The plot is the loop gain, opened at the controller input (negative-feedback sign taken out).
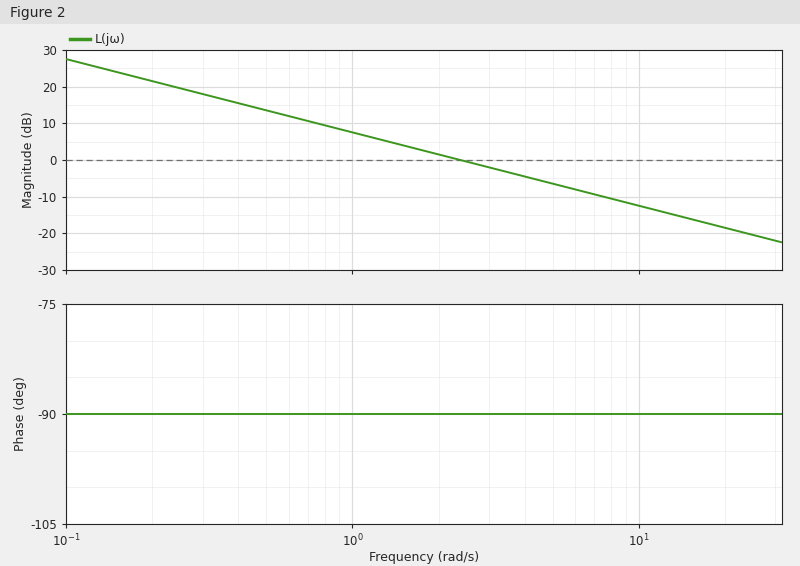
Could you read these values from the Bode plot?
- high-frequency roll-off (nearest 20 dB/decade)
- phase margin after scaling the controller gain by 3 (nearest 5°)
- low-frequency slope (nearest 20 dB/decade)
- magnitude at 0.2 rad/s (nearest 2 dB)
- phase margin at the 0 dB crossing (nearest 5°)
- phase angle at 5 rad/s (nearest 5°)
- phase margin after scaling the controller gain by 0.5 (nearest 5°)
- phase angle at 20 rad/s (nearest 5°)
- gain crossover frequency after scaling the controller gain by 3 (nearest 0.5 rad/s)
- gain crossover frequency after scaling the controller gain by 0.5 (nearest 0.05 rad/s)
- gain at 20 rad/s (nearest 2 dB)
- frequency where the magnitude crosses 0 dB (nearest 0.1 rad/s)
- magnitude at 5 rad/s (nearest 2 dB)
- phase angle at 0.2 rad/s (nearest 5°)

-20 dB/decade
90°
-20 dB/decade
22 dB
90°
-90°
90°
-90°
7.0 rad/s
1.20 rad/s
-18 dB
2.4 rad/s
-6 dB
-90°
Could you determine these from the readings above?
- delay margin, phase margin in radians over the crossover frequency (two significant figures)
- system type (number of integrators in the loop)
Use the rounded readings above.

0.65 s
1
